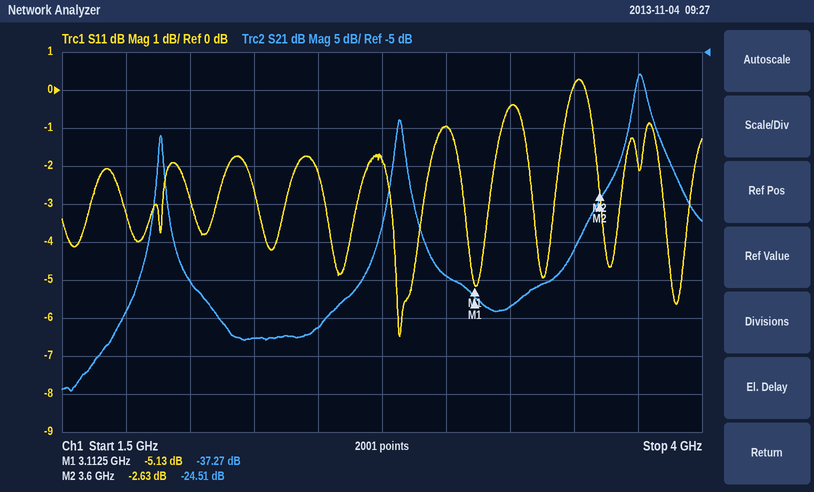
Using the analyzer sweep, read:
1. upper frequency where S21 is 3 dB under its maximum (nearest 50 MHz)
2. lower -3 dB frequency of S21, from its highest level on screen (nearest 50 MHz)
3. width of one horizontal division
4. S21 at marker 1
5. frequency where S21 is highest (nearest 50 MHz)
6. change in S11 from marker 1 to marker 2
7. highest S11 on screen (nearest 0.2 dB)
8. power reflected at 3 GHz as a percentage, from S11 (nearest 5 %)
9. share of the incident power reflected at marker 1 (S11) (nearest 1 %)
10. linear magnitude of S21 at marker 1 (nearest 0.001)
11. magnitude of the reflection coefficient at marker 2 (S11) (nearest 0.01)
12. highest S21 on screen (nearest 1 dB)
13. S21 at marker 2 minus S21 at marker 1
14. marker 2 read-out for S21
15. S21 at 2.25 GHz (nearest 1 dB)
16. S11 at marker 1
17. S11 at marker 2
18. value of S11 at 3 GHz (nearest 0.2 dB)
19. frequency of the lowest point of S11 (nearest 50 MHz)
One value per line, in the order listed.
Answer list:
3.80 GHz
3.75 GHz
250 MHz
-37.27 dB
3.75 GHz
2.50 dB
0.2 dB
80 %
31 %
0.014
0.74
-8 dB
12.76 dB
-24.51 dB
-43 dB
-5.13 dB
-2.63 dB
-1.0 dB
2.80 GHz
